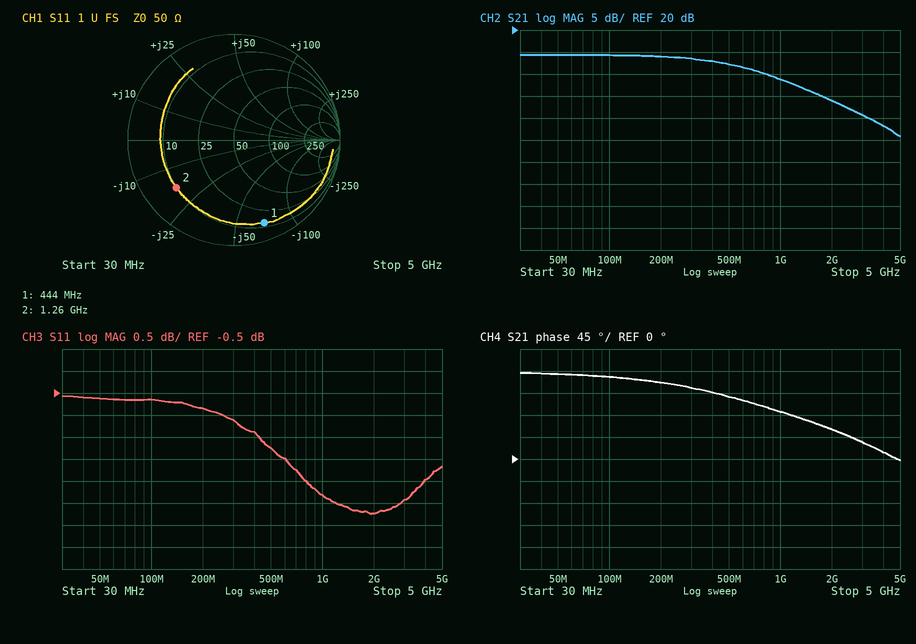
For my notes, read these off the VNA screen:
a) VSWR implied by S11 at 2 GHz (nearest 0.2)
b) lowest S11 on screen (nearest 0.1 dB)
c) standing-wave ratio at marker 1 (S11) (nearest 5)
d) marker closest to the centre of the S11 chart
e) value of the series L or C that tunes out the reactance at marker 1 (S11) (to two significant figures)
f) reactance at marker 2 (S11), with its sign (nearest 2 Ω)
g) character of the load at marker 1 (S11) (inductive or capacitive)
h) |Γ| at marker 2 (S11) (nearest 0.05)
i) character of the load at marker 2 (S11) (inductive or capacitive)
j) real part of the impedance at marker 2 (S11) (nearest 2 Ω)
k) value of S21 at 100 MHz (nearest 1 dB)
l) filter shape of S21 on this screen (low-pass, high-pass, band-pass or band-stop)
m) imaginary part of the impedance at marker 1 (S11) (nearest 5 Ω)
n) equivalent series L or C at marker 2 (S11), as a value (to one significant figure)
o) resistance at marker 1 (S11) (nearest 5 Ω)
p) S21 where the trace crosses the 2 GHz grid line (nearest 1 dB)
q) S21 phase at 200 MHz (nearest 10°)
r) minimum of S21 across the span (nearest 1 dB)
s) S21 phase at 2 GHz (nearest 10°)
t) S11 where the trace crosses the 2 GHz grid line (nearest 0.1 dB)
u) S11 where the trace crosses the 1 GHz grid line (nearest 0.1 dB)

5.4
-3.2 dB
10
marker 2
25 nH
-18 Ω
capacitive
0.70
capacitive
10 Ω
14 dB
low-pass
-70 Ω
7 pF
15 Ω
4 dB
160°
-4 dB
60°
-3.2 dB
-2.8 dB
